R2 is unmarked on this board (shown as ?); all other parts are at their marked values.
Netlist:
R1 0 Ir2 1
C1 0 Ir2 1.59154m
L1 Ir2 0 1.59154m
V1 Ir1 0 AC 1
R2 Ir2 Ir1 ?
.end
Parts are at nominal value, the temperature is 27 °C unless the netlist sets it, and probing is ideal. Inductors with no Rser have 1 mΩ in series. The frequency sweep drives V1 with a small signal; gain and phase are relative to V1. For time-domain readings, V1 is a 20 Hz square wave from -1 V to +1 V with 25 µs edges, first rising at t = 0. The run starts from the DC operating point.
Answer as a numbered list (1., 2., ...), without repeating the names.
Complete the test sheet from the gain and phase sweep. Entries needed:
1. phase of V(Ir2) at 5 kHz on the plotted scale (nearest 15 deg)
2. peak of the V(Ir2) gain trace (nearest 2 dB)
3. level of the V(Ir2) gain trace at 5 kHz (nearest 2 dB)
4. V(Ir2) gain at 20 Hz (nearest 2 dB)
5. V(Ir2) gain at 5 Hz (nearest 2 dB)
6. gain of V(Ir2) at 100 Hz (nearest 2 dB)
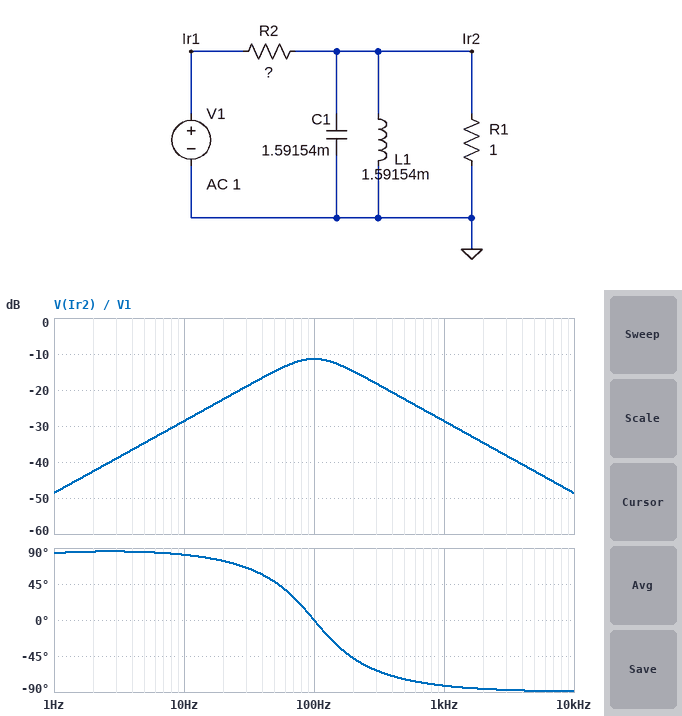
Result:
1. -90 deg
2. -12 dB
3. -42 dB
4. -22 dB
5. -34 dB
6. -12 dB
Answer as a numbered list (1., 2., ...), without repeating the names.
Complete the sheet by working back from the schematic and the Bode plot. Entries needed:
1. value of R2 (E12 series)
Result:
1. 2.7 Ω
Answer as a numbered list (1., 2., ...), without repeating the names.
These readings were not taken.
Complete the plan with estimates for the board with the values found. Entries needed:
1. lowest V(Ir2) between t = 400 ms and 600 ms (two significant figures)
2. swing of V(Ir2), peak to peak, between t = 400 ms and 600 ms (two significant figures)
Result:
1. -340 mV
2. 690 mV
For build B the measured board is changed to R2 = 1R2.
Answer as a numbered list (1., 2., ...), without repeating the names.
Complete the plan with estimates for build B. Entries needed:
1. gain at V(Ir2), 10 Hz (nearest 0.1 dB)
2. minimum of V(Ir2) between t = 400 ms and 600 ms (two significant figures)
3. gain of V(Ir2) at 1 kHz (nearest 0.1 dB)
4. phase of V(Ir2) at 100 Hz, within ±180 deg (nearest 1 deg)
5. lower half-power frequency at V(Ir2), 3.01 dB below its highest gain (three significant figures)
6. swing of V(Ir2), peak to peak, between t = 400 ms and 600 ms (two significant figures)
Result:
1. -21.7 dB
2. -650 mV
3. -21.6 dB
4. 0 deg
5. 44.0 Hz
6. 1.3 V
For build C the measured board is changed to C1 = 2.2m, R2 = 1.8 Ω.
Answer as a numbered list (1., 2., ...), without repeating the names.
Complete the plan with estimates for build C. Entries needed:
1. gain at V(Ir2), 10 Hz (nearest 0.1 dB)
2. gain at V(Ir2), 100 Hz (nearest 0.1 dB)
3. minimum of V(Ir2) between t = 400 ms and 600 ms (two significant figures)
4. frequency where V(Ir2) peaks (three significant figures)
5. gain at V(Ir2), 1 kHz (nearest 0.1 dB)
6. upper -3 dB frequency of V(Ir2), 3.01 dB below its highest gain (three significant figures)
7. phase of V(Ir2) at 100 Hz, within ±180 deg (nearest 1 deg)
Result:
1. -25.1 dB
2. -9.2 dB
3. -450 mV
4. 85.1 Hz
5. -27.9 dB
6. 158 Hz
7. -14 deg
